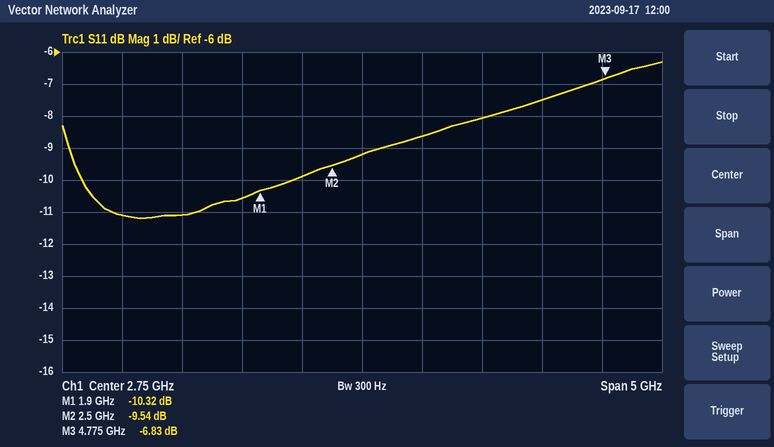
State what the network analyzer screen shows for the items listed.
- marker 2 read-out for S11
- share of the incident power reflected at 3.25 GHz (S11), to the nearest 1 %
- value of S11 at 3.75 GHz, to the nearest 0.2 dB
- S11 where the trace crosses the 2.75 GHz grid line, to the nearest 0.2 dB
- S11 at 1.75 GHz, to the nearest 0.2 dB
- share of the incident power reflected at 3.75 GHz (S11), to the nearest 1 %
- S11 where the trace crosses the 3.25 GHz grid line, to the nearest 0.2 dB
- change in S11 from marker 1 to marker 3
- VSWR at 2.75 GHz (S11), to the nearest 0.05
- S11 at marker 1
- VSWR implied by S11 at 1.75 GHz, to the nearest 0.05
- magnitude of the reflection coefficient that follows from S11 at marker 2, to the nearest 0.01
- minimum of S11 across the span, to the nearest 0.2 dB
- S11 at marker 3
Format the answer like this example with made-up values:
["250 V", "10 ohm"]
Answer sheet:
["-9.54 dB", "14 %", "-8.0 dB", "-9.2 dB", "-10.6 dB", "16 %", "-8.6 dB", "3.49 dB", "2.05", "-10.32 dB", "1.85", "0.33", "-11.2 dB", "-6.83 dB"]
